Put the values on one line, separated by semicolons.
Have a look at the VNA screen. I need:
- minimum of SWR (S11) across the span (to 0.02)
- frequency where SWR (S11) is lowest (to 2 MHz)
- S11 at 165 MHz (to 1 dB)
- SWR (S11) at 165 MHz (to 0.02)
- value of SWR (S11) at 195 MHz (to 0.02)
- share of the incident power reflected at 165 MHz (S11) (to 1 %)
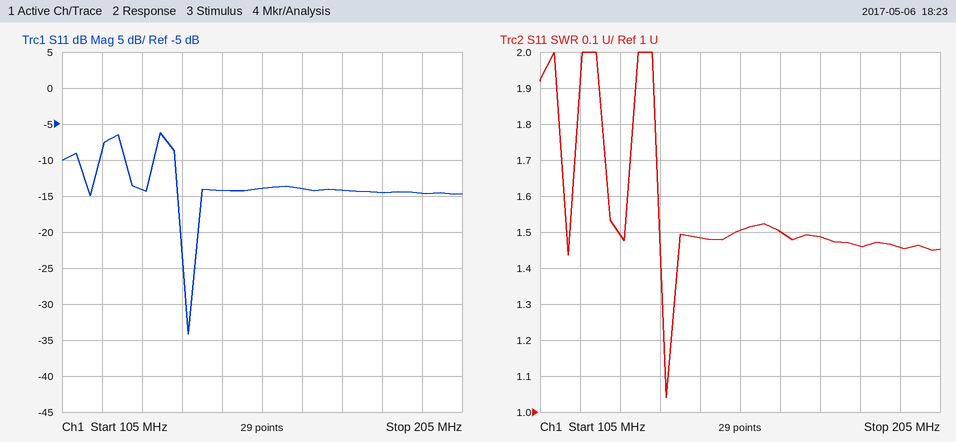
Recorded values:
1.04; 136 MHz; -14 dB; 1.50; 1.46; 4 %
